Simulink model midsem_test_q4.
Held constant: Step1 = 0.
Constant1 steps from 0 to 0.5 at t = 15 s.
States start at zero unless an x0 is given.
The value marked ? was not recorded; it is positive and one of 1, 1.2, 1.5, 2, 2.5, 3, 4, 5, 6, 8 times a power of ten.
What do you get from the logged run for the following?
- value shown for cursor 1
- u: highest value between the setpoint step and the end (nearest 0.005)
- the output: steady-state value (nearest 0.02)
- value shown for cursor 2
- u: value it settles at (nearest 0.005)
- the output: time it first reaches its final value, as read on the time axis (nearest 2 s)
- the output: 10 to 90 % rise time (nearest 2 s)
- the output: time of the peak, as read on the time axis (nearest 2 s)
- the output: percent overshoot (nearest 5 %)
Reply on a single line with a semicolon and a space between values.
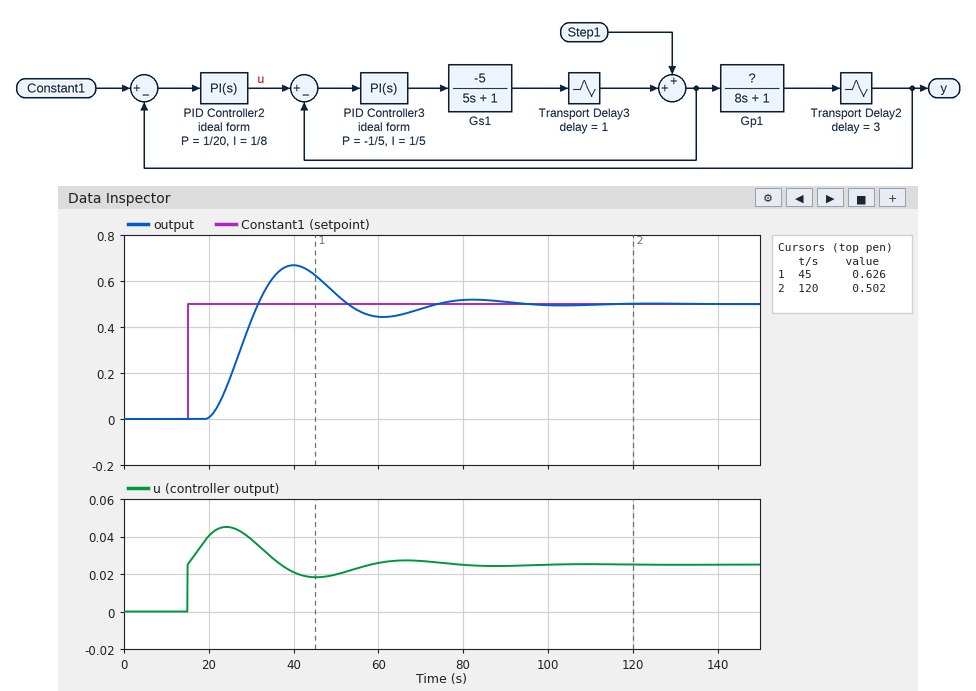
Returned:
0.626; 0.045; 0.50; 0.502; 0.025; 32 s; 8 s; 40 s; 35 %
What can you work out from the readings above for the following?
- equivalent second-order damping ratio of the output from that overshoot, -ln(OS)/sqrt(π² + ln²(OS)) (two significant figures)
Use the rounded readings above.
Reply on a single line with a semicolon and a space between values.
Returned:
0.32
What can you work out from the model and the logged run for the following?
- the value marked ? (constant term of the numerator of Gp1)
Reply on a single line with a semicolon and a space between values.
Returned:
20
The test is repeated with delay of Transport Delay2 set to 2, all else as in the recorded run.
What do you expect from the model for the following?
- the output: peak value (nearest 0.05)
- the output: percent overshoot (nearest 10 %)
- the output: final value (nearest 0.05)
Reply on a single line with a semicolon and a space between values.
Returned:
0.60; 20 %; 0.50
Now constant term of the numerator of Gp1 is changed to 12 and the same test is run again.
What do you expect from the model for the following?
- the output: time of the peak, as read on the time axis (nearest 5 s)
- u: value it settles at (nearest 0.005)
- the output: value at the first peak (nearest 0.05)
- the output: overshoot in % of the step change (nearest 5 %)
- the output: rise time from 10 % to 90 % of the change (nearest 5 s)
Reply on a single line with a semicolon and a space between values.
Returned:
50 s; 0.040; 0.55; 10 %; 15 s
